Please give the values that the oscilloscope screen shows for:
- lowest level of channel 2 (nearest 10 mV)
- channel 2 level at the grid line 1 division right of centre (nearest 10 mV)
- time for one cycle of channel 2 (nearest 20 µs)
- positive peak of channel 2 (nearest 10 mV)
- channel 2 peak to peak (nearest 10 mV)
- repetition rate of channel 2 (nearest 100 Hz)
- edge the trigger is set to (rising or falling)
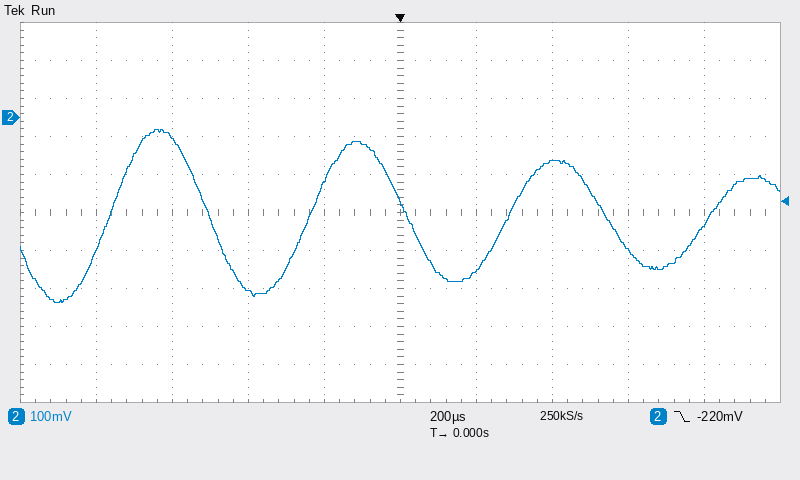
-490 mV
-400 mV
520 µs
-30 mV
460 mV
1.9 kHz
falling
